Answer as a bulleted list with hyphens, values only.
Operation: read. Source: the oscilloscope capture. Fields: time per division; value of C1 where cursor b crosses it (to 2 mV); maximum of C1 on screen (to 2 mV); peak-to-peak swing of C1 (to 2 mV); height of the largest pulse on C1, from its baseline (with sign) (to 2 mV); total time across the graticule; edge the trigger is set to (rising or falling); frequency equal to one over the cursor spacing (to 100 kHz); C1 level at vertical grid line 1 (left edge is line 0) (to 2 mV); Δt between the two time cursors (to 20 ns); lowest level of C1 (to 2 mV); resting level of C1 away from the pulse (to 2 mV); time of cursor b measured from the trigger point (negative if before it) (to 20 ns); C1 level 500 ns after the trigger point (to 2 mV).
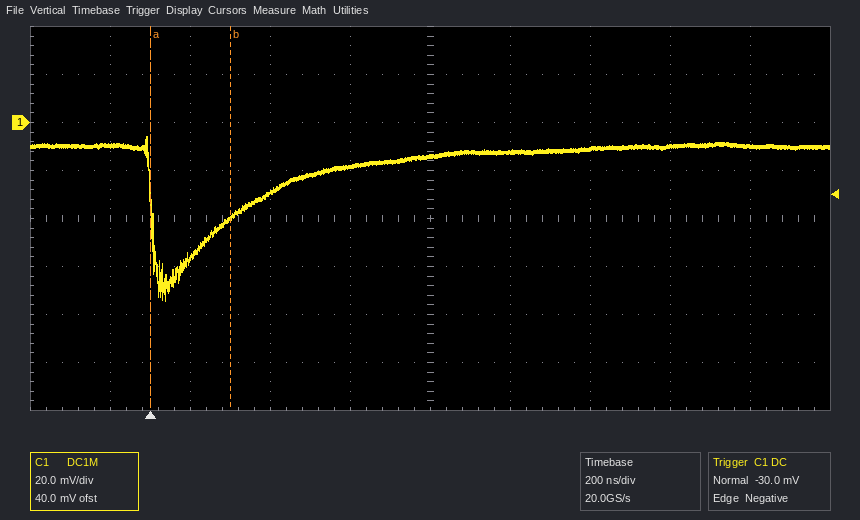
- 200 ns
- -40 mV
- -6 mV
- 68 mV
- -64 mV
- 2 µs
- falling
- 5.0 MHz
- -10 mV
- 200 ns
- -74 mV
- -10 mV
- +200 ns
- -18 mV
